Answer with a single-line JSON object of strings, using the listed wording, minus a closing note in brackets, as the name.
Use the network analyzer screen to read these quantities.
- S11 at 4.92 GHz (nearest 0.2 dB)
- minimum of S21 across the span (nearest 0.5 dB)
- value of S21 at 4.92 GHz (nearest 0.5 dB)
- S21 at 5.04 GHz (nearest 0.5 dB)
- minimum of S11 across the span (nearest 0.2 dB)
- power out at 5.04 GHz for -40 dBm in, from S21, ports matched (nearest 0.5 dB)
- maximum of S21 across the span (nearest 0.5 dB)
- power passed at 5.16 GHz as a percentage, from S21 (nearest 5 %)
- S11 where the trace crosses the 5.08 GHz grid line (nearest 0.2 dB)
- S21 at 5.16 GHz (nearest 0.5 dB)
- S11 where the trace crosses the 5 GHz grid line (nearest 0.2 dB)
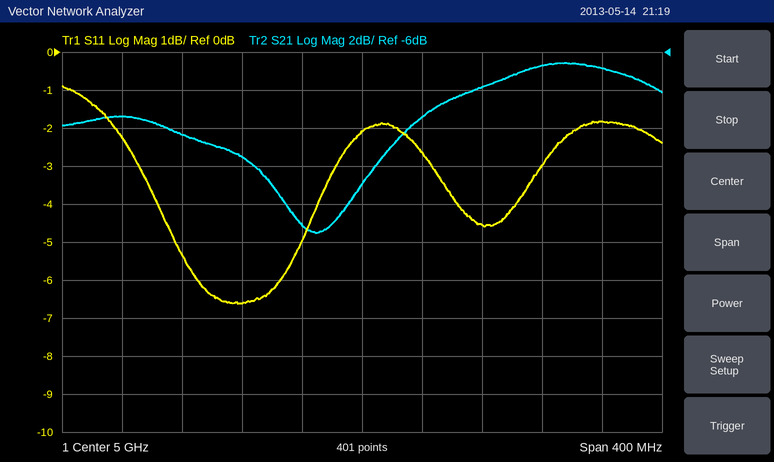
{"S11 at 4.92 GHz": "-6.6 dB", "minimum of S21 across the span": "-15.5 dB", "value of S21 at 4.92 GHz": "-11.5 dB", "S21 at 5.04 GHz": "-9.5 dB", "minimum of S11 across the span": "-6.6 dB", "power out at 5.04 GHz for -40 dBm in, from S21, ports matched": "-49.5 dBm", "maximum of S21 across the span": "-6.5 dB", "power passed at 5.16 GHz as a percentage, from S21": "20 %", "S11 where the trace crosses the 5.08 GHz grid line": "-4.6 dB", "S21 at 5.16 GHz": "-7.0 dB", "S11 where the trace crosses the 5 GHz grid line": "-2.0 dB"}
